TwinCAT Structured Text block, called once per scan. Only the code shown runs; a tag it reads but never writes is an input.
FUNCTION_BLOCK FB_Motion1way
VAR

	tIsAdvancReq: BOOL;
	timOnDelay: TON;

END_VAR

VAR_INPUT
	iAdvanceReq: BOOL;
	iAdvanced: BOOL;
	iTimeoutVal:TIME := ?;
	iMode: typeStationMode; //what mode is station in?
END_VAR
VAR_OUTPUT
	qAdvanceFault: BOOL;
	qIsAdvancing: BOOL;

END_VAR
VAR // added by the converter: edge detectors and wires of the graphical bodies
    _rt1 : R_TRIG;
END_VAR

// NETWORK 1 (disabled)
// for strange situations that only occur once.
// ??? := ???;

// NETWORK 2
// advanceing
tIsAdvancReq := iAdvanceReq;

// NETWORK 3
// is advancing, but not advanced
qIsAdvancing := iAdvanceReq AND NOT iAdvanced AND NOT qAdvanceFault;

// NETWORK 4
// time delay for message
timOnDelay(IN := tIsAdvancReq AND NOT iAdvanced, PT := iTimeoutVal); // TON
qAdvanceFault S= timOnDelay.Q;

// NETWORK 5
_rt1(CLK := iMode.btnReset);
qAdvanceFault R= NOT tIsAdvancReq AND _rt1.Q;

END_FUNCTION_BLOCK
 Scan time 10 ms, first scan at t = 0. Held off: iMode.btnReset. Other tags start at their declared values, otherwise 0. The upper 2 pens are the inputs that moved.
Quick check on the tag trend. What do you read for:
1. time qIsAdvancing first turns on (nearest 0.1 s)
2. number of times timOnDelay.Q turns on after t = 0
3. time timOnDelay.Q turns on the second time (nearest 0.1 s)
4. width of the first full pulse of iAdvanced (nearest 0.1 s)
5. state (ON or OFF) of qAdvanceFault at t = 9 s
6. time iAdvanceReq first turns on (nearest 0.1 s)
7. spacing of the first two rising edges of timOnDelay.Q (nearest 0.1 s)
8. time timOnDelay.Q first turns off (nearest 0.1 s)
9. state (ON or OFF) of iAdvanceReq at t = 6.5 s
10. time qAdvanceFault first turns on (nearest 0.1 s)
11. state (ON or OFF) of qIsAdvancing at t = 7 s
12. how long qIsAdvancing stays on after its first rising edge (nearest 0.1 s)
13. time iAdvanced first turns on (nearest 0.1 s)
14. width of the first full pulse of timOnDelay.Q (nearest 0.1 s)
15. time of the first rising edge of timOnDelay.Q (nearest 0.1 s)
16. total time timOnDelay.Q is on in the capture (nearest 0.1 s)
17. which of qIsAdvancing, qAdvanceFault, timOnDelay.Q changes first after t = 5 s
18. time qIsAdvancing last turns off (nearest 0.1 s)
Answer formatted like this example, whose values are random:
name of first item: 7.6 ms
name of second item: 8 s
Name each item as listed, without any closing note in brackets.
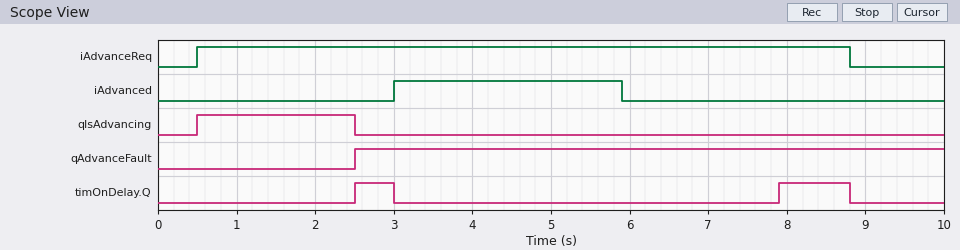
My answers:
time qIsAdvancing first turns on: 0.5 s
number of times timOnDelay.Q turns on after t = 0: 2
time timOnDelay.Q turns on the second time: 7.9 s
width of the first full pulse of iAdvanced: 2.9 s
state (ON or OFF) of qAdvanceFault at t = 9 s: ON
time iAdvanceReq first turns on: 0.5 s
spacing of the first two rising edges of timOnDelay.Q: 5.4 s
time timOnDelay.Q first turns off: 3.0 s
state (ON or OFF) of iAdvanceReq at t = 6.5 s: ON
time qAdvanceFault first turns on: 2.5 s
state (ON or OFF) of qIsAdvancing at t = 7 s: OFF
how long qIsAdvancing stays on after its first rising edge: 2.0 s
time iAdvanced first turns on: 3.0 s
width of the first full pulse of timOnDelay.Q: 0.5 s
time of the first rising edge of timOnDelay.Q: 2.5 s
total time timOnDelay.Q is on in the capture: 1.4 s
which of qIsAdvancing, qAdvanceFault, timOnDelay.Q changes first after t = 5 s: timOnDelay.Q
time qIsAdvancing last turns off: 2.5 s
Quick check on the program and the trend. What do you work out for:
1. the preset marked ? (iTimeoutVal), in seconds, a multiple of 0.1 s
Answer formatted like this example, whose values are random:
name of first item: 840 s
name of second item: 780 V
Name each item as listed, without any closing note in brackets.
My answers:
the preset marked ? (iTimeoutVal), in seconds, a multiple of 0.1 s: 2.0 s
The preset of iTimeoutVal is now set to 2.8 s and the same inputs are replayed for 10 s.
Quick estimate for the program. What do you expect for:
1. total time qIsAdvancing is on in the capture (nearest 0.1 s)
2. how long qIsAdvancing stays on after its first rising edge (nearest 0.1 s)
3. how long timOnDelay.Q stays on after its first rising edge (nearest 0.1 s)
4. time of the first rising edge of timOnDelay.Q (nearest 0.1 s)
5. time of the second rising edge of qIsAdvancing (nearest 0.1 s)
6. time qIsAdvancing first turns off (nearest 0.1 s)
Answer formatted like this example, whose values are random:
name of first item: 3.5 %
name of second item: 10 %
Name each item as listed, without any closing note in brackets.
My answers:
total time qIsAdvancing is on in the capture: 5.3 s
how long qIsAdvancing stays on after its first rising edge: 2.5 s
how long timOnDelay.Q stays on after its first rising edge: 0.1 s
time of the first rising edge of timOnDelay.Q: 8.7 s
time of the second rising edge of qIsAdvancing: 5.9 s
time qIsAdvancing first turns off: 3.0 s
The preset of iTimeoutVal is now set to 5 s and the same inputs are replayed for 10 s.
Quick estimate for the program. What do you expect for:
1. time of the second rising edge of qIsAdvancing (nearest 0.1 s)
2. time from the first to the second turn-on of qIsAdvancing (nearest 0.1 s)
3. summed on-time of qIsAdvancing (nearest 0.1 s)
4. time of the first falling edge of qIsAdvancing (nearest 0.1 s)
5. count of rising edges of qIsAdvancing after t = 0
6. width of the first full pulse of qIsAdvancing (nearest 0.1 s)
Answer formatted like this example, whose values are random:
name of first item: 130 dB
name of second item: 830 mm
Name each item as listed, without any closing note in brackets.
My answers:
time of the second rising edge of qIsAdvancing: 5.9 s
time from the first to the second turn-on of qIsAdvancing: 5.4 s
summed on-time of qIsAdvancing: 5.4 s
time of the first falling edge of qIsAdvancing: 3.0 s
count of rising edges of qIsAdvancing after t = 0: 2
width of the first full pulse of qIsAdvancing: 2.5 s
